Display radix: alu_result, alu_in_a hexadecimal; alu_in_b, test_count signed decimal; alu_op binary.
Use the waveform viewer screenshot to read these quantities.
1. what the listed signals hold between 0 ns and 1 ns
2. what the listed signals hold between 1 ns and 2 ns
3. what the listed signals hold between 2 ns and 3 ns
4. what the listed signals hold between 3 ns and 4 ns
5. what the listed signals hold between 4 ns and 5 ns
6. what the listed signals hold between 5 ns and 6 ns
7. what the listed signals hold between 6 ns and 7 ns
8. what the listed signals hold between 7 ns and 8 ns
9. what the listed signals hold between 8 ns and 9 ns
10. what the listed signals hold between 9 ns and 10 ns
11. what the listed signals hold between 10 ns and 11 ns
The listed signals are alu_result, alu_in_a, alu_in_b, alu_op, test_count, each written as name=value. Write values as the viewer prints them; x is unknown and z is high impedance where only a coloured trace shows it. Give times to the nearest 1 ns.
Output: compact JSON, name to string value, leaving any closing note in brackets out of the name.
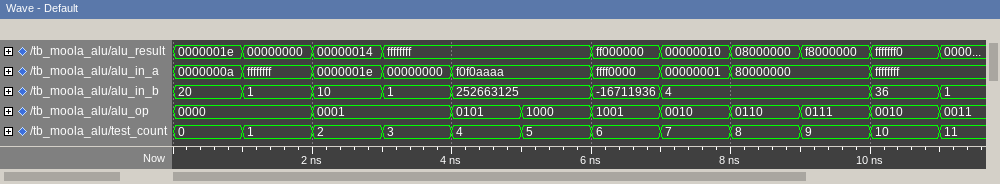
{"what the listed signals hold between 0 ns and 1 ns": "alu_result=0000001e, alu_in_a=0000000a, alu_in_b=20, alu_op=0000, test_count=0", "what the listed signals hold between 1 ns and 2 ns": "alu_result=00000000, alu_in_a=ffffffff, alu_in_b=1, alu_op=0000, test_count=1", "what the listed signals hold between 2 ns and 3 ns": "alu_result=00000014, alu_in_a=0000001e, alu_in_b=10, alu_op=0001, test_count=2", "what the listed signals hold between 3 ns and 4 ns": "alu_result=ffffffff, alu_in_a=00000000, alu_in_b=1, alu_op=0001, test_count=3", "what the listed signals hold between 4 ns and 5 ns": "alu_result=ffffffff, alu_in_a=f0f0aaaa, alu_in_b=252663125, alu_op=0101, test_count=4", "what the listed signals hold between 5 ns and 6 ns": "alu_result=ffffffff, alu_in_a=f0f0aaaa, alu_in_b=252663125, alu_op=1000, test_count=5", "what the listed signals hold between 6 ns and 7 ns": "alu_result=ff000000, alu_in_a=ffff0000, alu_in_b=-16711936, alu_op=1001, test_count=6", "what the listed signals hold between 7 ns and 8 ns": "alu_result=00000010, alu_in_a=00000001, alu_in_b=4, alu_op=0010, test_count=7", "what the listed signals hold between 8 ns and 9 ns": "alu_result=08000000, alu_in_a=80000000, alu_in_b=4, alu_op=0110, test_count=8", "what the listed signals hold between 9 ns and 10 ns": "alu_result=f8000000, alu_in_a=80000000, alu_in_b=4, alu_op=0111, test_count=9", "what the listed signals hold between 10 ns and 11 ns": "alu_result=fffffff0, alu_in_a=ffffffff, alu_in_b=36, alu_op=0010, test_count=10"}
